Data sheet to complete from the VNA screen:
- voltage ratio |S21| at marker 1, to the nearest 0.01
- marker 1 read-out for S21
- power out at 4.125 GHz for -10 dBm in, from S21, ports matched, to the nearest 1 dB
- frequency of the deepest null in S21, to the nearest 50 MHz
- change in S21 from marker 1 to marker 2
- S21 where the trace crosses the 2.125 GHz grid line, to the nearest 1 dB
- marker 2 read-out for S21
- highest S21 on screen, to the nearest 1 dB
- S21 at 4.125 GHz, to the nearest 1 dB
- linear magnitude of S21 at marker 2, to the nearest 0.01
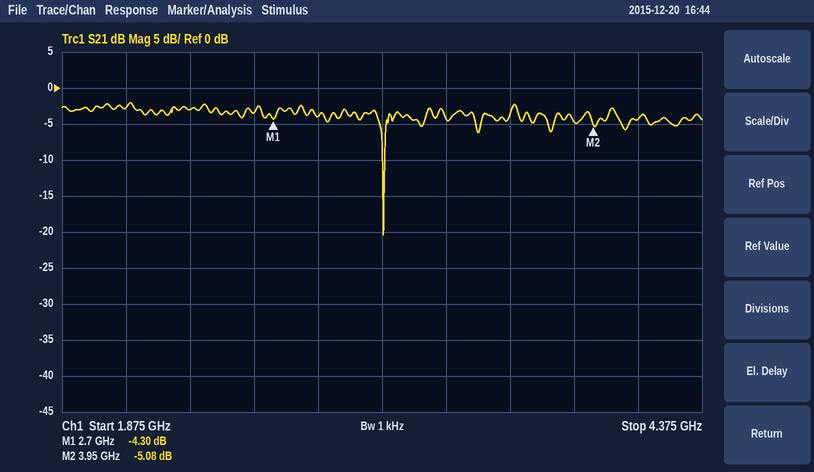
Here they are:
0.61
-4.30 dB
-14 dBm
3.15 GHz
-0.78 dB
-3 dB
-5.08 dB
-2 dB
-4 dB
0.56
